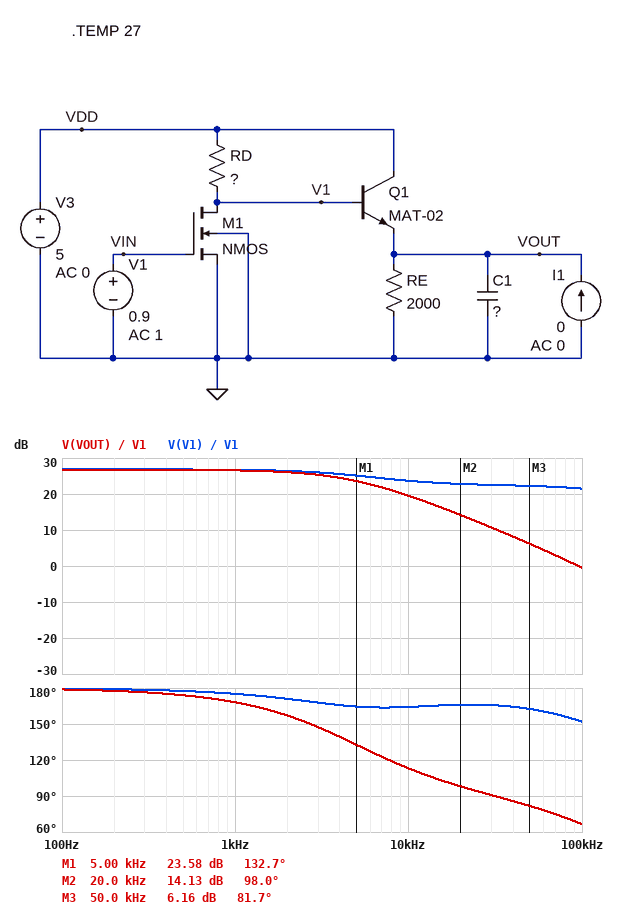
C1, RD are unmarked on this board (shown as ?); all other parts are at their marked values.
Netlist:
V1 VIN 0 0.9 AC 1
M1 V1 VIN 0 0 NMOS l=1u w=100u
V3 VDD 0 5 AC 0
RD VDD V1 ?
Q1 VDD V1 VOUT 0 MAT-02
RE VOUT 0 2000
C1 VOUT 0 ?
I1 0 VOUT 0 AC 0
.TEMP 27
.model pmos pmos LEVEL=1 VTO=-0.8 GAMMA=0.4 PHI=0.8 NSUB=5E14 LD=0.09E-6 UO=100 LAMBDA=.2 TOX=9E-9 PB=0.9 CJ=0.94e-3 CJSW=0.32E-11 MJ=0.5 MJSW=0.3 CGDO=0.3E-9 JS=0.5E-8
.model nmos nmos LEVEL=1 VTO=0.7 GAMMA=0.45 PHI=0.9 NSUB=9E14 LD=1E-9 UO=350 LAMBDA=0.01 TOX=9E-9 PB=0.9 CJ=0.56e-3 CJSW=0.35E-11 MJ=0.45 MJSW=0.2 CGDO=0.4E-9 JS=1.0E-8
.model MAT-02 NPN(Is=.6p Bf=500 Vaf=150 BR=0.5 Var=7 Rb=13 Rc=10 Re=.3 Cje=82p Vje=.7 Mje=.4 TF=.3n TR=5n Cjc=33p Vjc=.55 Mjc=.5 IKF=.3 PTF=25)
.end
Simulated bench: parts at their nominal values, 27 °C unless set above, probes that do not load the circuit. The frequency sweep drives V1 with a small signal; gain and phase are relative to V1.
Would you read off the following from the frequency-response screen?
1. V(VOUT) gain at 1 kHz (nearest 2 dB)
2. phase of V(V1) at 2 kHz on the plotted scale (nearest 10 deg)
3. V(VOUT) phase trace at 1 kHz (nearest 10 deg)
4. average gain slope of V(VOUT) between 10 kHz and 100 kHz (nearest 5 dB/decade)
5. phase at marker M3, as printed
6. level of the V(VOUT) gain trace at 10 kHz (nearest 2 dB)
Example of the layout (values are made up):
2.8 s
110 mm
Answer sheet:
26 dB
170 deg
170 deg
-20 dB/decade
81.7 deg
20 dB
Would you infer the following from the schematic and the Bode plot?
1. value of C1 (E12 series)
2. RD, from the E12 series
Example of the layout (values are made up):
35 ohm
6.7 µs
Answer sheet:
820 nF
8.2 kΩ
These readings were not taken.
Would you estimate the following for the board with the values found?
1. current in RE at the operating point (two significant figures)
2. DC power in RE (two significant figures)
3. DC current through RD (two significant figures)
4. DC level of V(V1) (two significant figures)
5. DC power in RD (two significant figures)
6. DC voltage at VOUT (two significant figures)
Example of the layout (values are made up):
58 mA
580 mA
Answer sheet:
1.1 mA
2.3 mW
280 µA
2.7 V
640 µW
2.2 V
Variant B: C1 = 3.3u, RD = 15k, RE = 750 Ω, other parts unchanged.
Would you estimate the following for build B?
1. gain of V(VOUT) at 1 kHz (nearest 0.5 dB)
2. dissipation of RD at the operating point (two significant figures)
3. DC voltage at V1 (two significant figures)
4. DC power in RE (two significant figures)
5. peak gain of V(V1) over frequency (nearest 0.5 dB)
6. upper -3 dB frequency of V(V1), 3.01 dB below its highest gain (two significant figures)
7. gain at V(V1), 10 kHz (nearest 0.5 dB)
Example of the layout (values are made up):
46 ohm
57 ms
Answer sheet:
25.5 dB
1.1 mW
910 mV
190 µW
31.5 dB
1.8 kHz
28.0 dB
